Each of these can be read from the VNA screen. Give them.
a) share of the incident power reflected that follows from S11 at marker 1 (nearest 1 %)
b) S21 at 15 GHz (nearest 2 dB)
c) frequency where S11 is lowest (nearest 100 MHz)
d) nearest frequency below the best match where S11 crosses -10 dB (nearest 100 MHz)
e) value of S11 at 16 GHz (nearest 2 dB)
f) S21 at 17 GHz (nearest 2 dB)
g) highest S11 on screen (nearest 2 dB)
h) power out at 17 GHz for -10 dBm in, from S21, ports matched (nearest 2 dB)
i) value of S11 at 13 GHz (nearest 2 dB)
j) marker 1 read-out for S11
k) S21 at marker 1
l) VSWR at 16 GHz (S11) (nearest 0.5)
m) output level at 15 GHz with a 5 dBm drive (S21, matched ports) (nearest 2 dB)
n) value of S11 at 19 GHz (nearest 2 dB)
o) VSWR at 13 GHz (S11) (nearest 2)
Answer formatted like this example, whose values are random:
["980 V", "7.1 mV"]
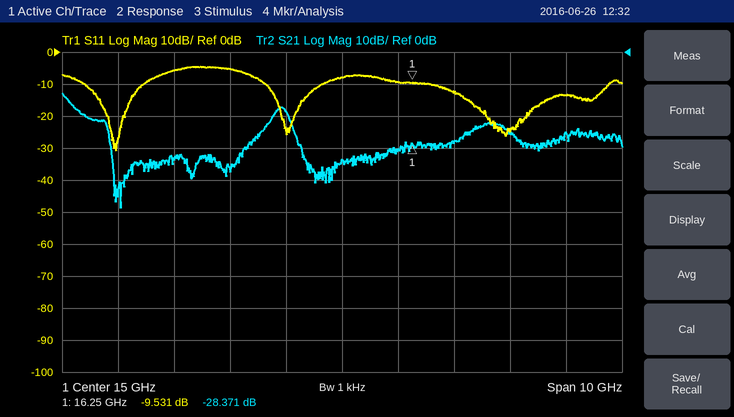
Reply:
["11 %", "-34 dB", "11.0 GHz", "10.4 GHz", "-10 dB", "-28 dB", "-4 dB", "-38 dBm", "-6 dB", "-9.531 dB", "-28.371 dB", "2.0", "-28 dBm", "-14 dB", "4"]
